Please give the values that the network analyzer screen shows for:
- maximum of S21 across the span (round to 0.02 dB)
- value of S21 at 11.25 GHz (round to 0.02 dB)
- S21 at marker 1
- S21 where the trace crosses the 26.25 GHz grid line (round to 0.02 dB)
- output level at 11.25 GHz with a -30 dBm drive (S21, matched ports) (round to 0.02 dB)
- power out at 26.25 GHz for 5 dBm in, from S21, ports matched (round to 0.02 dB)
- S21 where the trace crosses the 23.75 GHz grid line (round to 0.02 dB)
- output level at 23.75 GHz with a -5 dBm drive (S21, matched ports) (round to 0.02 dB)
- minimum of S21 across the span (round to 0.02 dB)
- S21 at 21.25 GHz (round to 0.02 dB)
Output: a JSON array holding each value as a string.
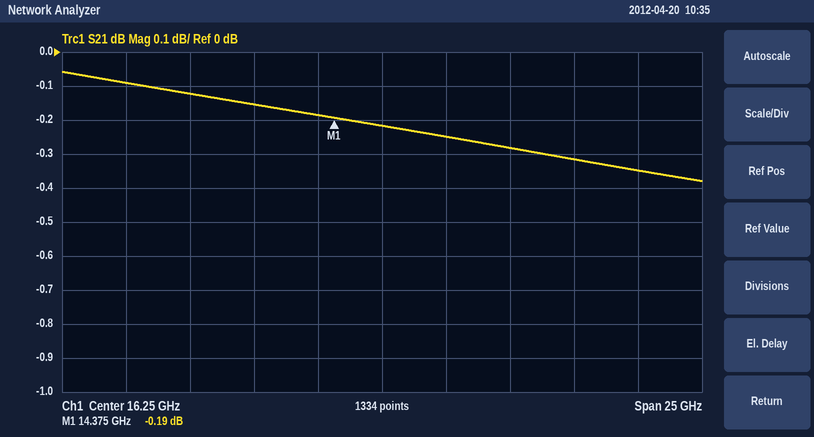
["-0.06 dB", "-0.16 dB", "-0.19 dB", "-0.34 dB", "-30.16 dBm", "4.66 dBm", "-0.32 dB", "-5.32 dBm", "-0.38 dB", "-0.28 dB"]
